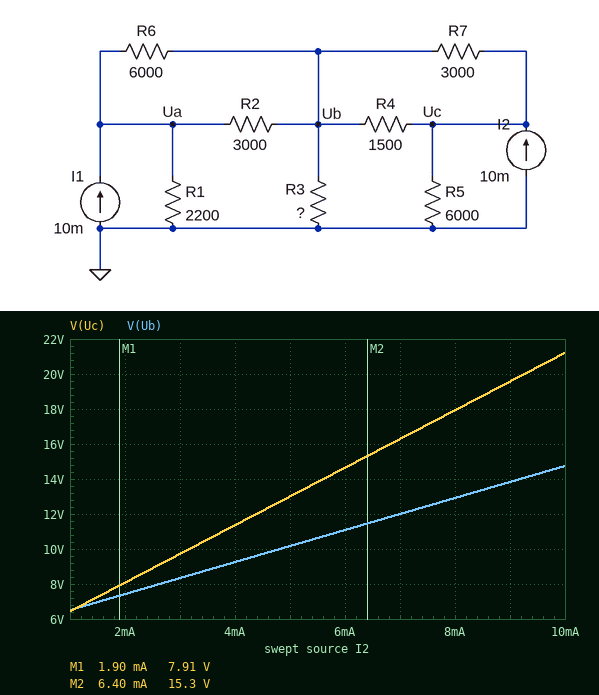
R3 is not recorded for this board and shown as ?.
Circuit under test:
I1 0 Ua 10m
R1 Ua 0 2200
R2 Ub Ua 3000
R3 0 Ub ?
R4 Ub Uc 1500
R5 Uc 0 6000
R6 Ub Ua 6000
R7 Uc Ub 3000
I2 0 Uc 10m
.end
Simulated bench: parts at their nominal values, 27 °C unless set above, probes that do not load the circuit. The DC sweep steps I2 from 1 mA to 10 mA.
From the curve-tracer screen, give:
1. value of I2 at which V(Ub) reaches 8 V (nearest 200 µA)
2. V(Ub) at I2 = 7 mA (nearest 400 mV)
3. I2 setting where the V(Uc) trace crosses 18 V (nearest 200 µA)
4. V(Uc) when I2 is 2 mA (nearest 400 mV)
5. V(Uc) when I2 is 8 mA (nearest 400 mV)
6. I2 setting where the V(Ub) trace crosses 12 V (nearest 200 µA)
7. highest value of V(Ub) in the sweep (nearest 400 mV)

2.6 mA
12.0 V
8.0 mA
8.0 V
18.0 V
7.0 mA
14.8 V
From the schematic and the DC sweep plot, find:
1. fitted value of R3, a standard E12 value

1.8 kΩ
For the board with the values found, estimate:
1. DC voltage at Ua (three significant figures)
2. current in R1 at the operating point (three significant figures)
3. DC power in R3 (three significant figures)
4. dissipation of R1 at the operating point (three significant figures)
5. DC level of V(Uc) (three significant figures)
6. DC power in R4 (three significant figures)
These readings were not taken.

18.2 V
8.27 mA
121 mW
151 mW
21.2 V
27.9 mW
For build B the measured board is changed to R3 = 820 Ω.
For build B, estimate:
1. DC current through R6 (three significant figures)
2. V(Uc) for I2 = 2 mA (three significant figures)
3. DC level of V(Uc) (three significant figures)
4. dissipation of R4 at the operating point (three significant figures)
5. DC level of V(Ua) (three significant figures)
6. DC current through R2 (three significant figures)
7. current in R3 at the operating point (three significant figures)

1.06 mA
5.44 V
16.0 V
35.9 mW
15.0 V
2.12 mA
10.5 mA
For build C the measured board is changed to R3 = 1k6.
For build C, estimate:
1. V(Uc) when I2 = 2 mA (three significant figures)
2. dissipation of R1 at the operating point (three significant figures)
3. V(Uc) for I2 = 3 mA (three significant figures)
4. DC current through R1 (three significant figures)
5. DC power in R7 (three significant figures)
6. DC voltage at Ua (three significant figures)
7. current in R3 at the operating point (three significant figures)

7.64 V
142 mW
9.23 V
8.03 mA
14.6 mW
17.7 V
8.58 mA
